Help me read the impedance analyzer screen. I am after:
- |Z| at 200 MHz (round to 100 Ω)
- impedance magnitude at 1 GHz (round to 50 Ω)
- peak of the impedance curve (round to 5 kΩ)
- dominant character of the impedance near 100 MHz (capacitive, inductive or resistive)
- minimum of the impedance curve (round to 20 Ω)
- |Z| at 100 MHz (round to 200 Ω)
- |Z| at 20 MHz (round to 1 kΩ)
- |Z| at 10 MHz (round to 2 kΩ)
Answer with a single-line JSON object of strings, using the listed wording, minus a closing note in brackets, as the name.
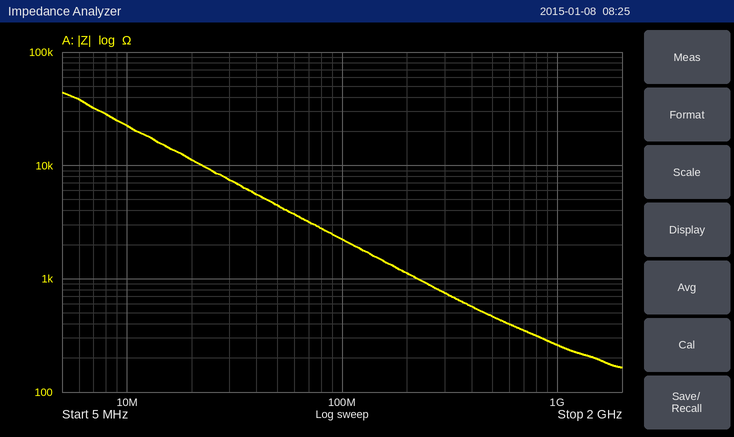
{"|Z| at 200 MHz": "1.1 kΩ", "impedance magnitude at 1 GHz": "250 Ω", "peak of the impedance curve": "45 kΩ", "dominant character of the impedance near 100 MHz": "capacitive", "minimum of the impedance curve": "160 Ω", "|Z| at 100 MHz": "2.2 kΩ", "|Z| at 20 MHz": "11 kΩ", "|Z| at 10 MHz": "22 kΩ"}
